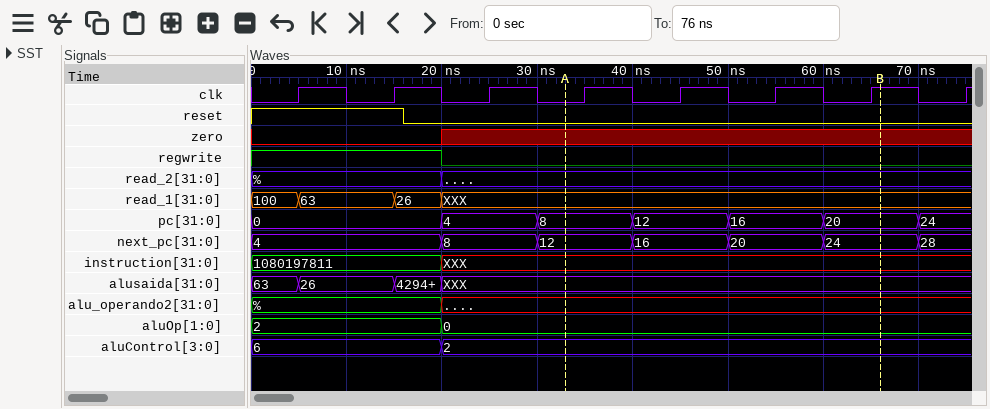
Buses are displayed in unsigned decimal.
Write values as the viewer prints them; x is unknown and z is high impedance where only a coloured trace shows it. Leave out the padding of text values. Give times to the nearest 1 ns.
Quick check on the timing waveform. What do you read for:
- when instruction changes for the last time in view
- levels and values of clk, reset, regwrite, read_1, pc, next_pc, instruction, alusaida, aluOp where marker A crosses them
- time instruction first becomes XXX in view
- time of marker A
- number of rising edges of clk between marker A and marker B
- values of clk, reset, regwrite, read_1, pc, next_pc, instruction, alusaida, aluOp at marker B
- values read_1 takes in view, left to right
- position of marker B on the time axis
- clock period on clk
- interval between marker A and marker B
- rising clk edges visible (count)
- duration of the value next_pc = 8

20 ns
clk=0, reset=0, regwrite=0, read_1=XXX, pc=8, next_pc=12, instruction=XXX, alusaida=XXX, aluOp=0
20 ns
33 ns
4
clk=1, reset=0, regwrite=0, read_1=XXX, pc=20, next_pc=24, instruction=XXX, alusaida=XXX, aluOp=0
100, 63, 26, XXX
66 ns
10 ns
33 ns
8
10 ns
